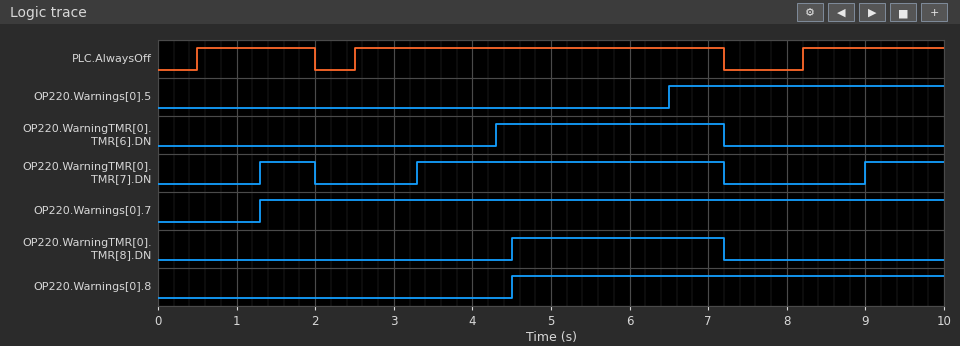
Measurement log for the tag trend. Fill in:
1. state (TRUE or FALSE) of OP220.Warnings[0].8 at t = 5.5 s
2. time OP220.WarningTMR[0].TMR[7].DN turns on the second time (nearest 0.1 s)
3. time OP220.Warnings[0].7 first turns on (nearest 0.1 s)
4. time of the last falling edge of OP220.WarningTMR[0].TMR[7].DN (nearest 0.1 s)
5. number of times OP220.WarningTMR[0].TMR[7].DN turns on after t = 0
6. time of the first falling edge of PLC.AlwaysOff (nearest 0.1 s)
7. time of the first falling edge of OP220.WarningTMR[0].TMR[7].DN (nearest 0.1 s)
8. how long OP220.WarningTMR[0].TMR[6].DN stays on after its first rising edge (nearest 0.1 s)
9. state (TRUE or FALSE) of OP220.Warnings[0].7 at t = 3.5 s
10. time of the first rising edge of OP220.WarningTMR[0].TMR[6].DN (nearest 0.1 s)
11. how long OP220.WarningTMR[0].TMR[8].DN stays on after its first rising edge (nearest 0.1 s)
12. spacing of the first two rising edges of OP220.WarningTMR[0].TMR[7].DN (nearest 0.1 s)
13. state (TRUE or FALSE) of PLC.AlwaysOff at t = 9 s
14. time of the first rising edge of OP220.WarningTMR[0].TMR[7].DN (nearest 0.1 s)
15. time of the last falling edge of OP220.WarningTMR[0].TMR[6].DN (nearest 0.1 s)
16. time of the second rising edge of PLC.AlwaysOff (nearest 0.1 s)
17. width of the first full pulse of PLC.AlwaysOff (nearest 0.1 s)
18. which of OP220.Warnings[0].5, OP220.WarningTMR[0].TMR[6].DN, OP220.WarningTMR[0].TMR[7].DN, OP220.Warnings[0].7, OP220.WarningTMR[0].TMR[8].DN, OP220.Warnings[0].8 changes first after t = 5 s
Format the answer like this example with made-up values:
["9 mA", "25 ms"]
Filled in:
["TRUE", "3.3 s", "1.3 s", "7.2 s", "3", "2.0 s", "2.0 s", "2.9 s", "TRUE", "4.3 s", "2.7 s", "2.0 s", "TRUE", "1.3 s", "7.2 s", "2.5 s", "1.5 s", "OP220.Warnings[0].5"]
